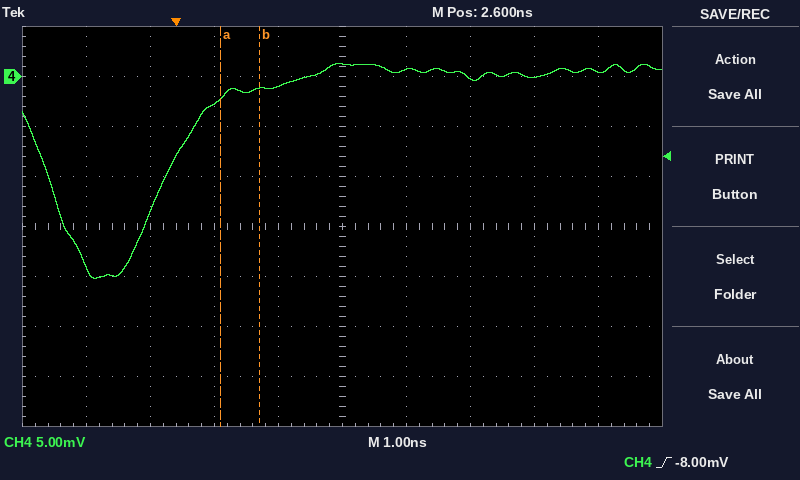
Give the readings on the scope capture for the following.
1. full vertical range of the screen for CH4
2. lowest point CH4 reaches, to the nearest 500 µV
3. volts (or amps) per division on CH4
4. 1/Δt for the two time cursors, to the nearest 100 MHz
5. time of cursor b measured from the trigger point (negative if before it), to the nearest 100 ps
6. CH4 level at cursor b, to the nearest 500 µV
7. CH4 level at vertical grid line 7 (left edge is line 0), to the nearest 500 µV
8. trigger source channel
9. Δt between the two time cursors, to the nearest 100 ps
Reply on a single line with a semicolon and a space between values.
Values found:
40 mV; -20.0 mV; 5 mV; 1.7 GHz; +1.3 ns; -1.0 mV; 0.0 mV; CH4; 600 ps
